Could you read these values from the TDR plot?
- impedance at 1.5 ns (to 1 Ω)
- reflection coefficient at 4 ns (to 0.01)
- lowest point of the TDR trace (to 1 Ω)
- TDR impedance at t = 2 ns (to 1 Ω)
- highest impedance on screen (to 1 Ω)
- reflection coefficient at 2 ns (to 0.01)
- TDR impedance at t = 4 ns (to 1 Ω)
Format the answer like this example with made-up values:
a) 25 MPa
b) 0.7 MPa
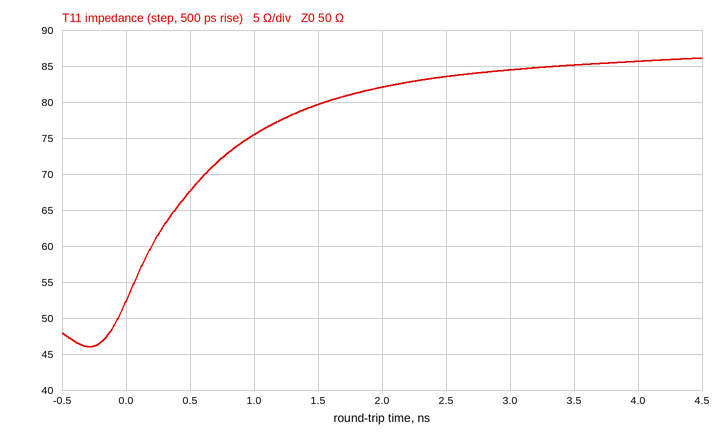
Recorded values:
a) 80 Ω
b) +0.26
c) 46 Ω
d) 82 Ω
e) 86 Ω
f) +0.24
g) 86 Ω
